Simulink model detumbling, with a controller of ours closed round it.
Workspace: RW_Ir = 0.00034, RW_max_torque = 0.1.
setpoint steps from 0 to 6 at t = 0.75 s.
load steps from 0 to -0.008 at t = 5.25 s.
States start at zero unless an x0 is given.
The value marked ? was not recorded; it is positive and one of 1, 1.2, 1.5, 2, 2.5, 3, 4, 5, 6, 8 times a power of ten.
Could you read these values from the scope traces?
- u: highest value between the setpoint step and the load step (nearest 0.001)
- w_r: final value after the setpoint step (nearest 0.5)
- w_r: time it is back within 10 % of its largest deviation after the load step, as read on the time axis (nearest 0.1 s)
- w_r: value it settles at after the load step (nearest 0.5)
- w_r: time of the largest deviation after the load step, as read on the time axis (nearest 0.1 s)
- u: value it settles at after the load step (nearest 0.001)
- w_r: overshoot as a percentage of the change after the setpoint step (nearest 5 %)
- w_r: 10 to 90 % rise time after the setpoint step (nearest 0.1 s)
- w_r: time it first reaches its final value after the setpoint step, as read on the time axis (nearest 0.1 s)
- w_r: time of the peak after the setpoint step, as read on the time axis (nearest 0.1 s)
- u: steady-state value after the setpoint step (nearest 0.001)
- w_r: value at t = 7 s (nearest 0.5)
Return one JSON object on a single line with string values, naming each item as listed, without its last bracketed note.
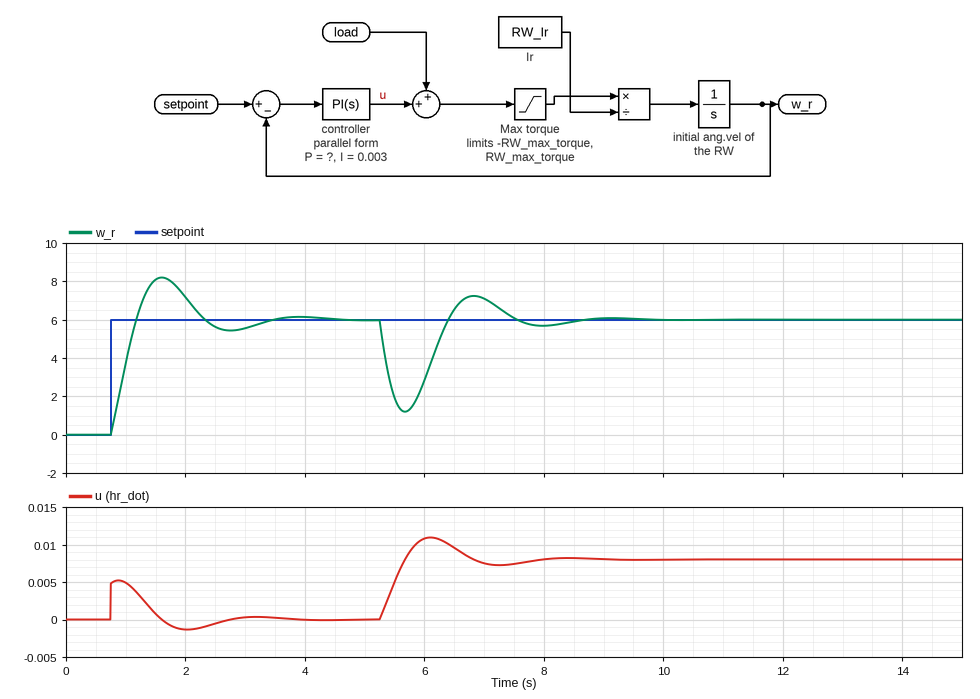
{"u: highest value between the setpoint step and the load step": "0.005", "w_r: final value after the setpoint step": "6.0", "w_r: time it is back within 10 % of its largest deviation after the load step, as read on the time axis": "7.3 s", "w_r: value it settles at after the load step": "6.0", "w_r: time of the largest deviation after the load step, as read on the time axis": "5.7 s", "u: value it settles at after the load step": "0.008", "w_r: overshoot as a percentage of the change after the setpoint step": "35 %", "w_r: 10 to 90 % rise time after the setpoint step": "0.3 s", "w_r: time it first reaches its final value after the setpoint step, as read on the time axis": "1.2 s", "w_r: time of the peak after the setpoint step, as read on the time axis": "1.6 s", "u: steady-state value after the setpoint step": "0.000", "w_r: value at t = 7 s": "7.0"}
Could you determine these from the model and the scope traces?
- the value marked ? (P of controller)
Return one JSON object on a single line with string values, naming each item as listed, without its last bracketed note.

{"the value marked ?": "0.0008"}
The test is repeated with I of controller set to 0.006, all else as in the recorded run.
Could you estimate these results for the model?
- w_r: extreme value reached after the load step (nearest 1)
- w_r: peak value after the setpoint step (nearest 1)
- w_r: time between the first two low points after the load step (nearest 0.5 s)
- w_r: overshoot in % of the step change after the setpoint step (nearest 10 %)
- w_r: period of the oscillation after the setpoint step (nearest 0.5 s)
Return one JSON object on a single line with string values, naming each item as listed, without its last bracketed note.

{"w_r: extreme value reached after the load step": "2", "w_r: peak value after the setpoint step": "9", "w_r: time between the first two low points after the load step": "1.5 s", "w_r: overshoot in % of the step change after the setpoint step": "50 %", "w_r: period of the oscillation after the setpoint step": "1.5 s"}
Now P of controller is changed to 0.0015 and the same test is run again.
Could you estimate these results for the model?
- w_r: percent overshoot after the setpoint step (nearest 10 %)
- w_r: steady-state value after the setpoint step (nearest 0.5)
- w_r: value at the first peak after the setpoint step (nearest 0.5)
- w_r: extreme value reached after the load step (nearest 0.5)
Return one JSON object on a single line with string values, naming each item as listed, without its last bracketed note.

{"w_r: percent overshoot after the setpoint step": "20 %", "w_r: steady-state value after the setpoint step": "6.0", "w_r: value at the first peak after the setpoint step": "7.0", "w_r: extreme value reached after the load step": "2.5"}
